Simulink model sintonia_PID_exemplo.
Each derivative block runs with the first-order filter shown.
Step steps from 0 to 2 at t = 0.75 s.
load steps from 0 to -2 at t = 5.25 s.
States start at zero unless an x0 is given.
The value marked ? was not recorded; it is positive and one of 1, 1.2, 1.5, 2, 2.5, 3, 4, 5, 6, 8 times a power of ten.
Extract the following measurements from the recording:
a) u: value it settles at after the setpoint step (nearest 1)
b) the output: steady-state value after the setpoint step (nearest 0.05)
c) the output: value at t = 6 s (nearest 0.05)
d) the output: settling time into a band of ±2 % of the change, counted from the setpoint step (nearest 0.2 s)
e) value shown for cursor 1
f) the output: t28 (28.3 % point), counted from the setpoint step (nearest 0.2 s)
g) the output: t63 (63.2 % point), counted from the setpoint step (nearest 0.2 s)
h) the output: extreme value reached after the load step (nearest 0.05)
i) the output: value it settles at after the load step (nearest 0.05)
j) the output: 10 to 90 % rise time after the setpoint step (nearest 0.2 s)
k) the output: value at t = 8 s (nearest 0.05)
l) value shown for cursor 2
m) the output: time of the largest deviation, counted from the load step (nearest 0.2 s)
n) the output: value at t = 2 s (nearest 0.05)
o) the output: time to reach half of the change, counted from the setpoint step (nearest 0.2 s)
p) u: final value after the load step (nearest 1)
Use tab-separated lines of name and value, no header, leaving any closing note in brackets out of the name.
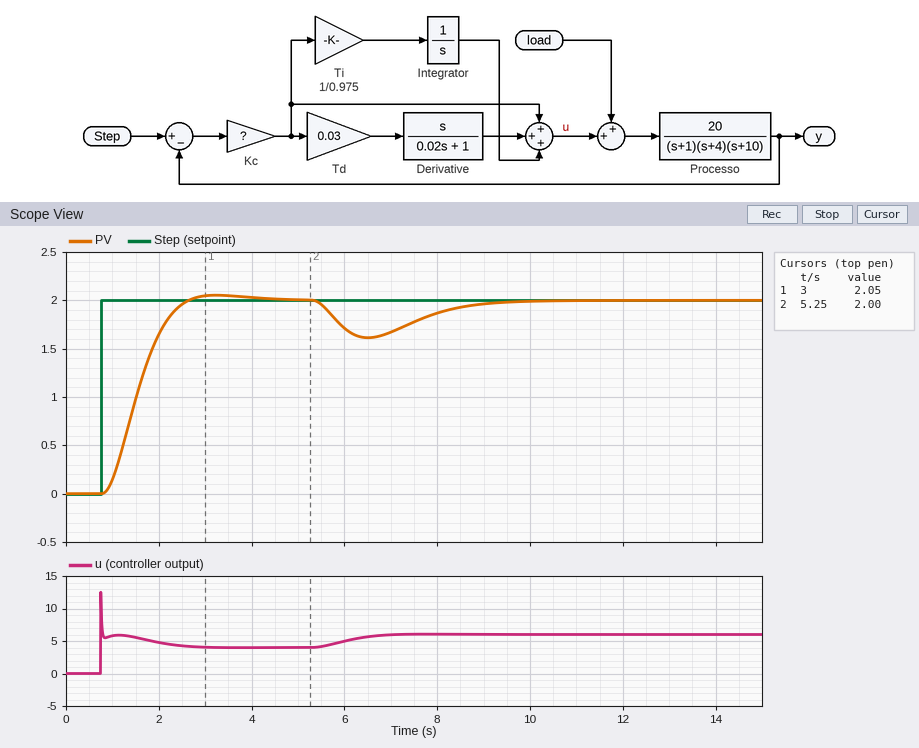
u: value it settles at after the setpoint step	4
the output: steady-state value after the setpoint step	2.00
the output: value at t = 6 s	1.70
the output: settling time into a band of ±2 % of the change, counted from the setpoint step	3.0 s
value shown for cursor 1	2.05
the output: t28 (28.3 % point), counted from the setpoint step	0.6 s
the output: t63 (63.2 % point), counted from the setpoint step	1.0 s
the output: extreme value reached after the load step	1.60
the output: value it settles at after the load step	2.00
the output: 10 to 90 % rise time after the setpoint step	1.2 s
the output: value at t = 8 s	1.85
value shown for cursor 2	2.00
the output: time of the largest deviation, counted from the load step	1.2 s
the output: value at t = 2 s	1.65
the output: time to reach half of the change, counted from the setpoint step	0.8 s
u: final value after the load step	6
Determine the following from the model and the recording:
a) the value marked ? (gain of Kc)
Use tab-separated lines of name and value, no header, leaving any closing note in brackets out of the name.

the value marked ?	2.5
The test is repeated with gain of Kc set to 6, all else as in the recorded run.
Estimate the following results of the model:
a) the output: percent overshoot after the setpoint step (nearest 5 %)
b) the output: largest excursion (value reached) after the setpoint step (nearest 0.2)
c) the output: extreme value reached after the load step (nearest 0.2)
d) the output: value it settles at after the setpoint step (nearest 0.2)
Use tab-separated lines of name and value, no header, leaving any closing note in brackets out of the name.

the output: percent overshoot after the setpoint step	20 %
the output: largest excursion (value reached) after the setpoint step	2.4
the output: extreme value reached after the load step	1.8
the output: value it settles at after the setpoint step	2.0
